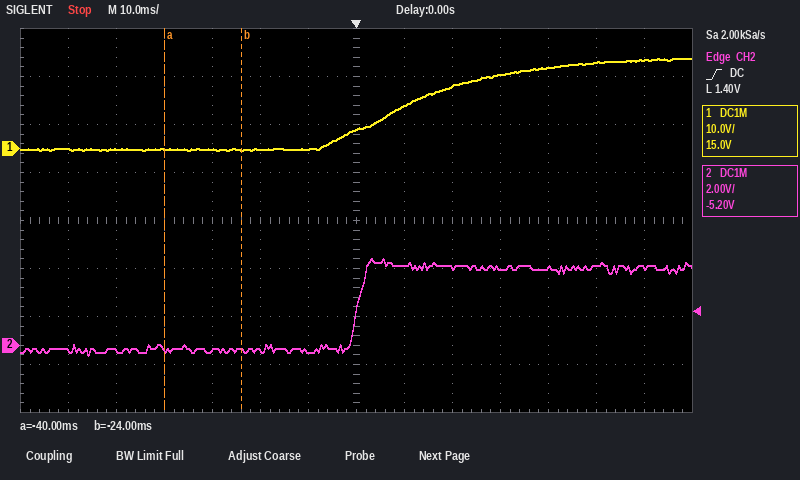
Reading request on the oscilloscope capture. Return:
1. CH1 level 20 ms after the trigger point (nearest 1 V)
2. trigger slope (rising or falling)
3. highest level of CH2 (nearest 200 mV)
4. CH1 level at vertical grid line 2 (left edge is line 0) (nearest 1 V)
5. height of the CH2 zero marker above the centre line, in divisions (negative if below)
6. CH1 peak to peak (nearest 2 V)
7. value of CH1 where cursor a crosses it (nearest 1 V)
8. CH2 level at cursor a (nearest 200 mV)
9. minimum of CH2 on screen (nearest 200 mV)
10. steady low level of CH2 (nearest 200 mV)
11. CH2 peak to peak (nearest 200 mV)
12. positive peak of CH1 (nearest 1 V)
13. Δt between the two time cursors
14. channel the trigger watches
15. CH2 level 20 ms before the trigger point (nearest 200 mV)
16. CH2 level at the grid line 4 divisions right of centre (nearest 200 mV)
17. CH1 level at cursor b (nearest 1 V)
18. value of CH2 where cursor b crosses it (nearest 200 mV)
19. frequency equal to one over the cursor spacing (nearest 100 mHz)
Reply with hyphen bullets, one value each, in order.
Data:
- 13 V
- rising
- 3.6 V
- 0 V
- -2.6 div
- 20 V
- 0 V
- -200 mV
- -400 mV
- -200 mV
- 4.0 V
- 19 V
- 16 ms
- CH2
- -200 mV
- 3.2 V
- 0 V
- -200 mV
- 62.5 Hz
